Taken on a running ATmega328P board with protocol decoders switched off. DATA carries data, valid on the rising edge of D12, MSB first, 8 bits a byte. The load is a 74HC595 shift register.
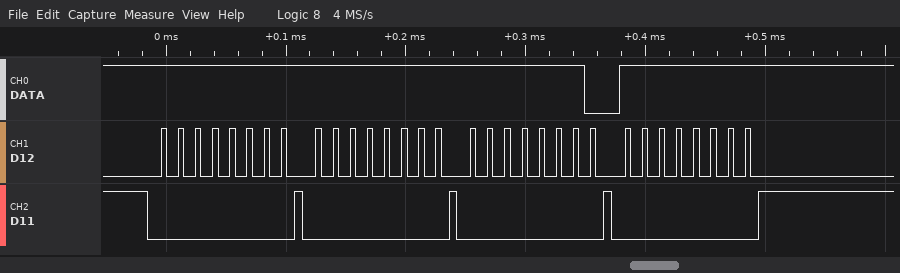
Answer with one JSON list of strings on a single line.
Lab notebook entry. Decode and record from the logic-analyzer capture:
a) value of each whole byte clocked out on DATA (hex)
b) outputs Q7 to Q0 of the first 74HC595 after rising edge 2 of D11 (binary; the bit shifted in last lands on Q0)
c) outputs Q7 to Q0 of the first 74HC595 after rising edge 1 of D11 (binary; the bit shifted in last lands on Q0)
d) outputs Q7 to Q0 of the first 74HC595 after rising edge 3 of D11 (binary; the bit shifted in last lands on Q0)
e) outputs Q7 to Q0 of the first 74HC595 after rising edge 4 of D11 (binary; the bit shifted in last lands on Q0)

["FF FF FE FF", "11111111", "11111111", "11111110", "11111111"]
